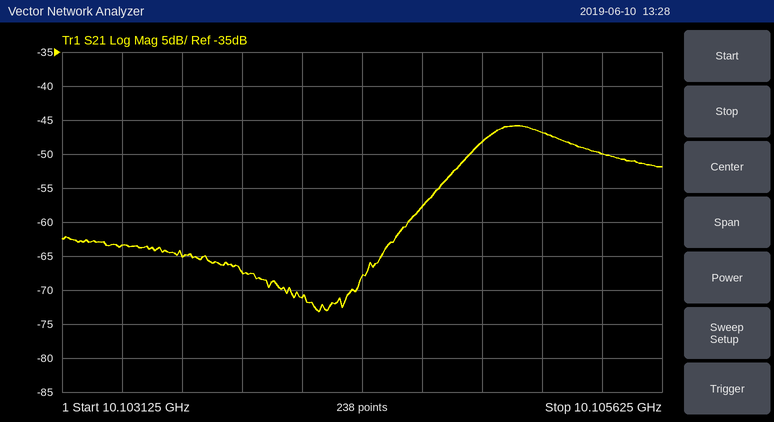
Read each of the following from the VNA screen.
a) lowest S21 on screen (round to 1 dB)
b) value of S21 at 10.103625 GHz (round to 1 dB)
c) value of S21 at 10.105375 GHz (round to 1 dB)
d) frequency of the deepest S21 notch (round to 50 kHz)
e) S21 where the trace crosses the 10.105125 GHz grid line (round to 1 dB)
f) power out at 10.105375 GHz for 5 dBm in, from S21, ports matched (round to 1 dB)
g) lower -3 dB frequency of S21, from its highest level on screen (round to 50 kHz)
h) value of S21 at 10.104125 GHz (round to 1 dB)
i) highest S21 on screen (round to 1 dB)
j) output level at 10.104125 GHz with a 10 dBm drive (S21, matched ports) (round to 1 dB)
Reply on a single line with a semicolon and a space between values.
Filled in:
-73 dB; -65 dB; -50 dB; 10.10420 GHz; -47 dB; -45 dBm; 10.10485 GHz; -71 dB; -46 dB; -61 dBm
